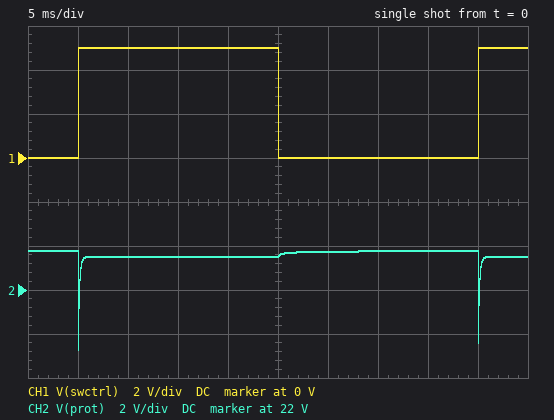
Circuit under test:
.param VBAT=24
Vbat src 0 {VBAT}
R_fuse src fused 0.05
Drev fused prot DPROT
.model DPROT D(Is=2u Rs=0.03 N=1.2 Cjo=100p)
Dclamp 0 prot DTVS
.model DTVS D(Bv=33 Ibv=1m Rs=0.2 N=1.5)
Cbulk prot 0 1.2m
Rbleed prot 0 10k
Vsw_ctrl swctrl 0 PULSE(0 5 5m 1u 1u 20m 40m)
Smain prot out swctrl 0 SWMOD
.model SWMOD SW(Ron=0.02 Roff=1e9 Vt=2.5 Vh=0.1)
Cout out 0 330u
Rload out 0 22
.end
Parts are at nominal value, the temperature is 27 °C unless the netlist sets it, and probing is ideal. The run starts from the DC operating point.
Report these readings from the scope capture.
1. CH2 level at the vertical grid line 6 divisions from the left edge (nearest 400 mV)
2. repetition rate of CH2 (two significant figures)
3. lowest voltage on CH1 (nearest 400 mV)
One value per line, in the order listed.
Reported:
23.6 V
25 Hz
0 V
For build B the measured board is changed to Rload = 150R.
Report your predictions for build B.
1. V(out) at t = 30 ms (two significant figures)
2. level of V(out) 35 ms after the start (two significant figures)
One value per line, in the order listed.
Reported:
21 V
19 V
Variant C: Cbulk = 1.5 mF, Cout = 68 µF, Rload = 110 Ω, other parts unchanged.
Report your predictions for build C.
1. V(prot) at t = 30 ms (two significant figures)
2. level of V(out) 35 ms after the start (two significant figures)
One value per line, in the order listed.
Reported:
24 V
6.2 V
